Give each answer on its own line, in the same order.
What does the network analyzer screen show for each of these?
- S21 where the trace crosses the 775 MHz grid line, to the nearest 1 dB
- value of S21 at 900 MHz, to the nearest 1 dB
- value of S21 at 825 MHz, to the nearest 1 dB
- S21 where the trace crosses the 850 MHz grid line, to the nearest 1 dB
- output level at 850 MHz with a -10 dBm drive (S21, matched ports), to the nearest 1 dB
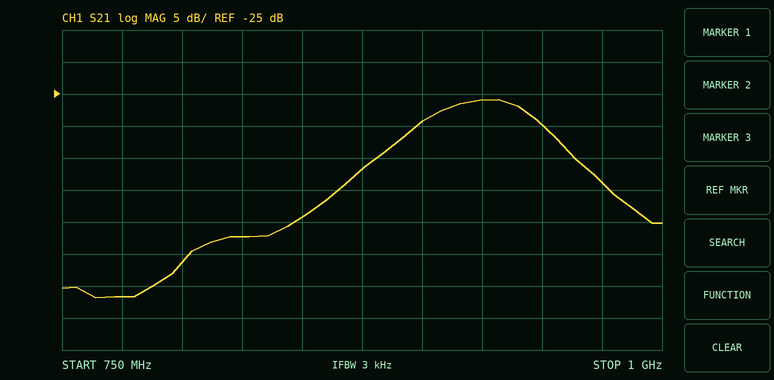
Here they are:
-57 dB
-29 dB
-47 dB
-44 dB
-54 dBm
